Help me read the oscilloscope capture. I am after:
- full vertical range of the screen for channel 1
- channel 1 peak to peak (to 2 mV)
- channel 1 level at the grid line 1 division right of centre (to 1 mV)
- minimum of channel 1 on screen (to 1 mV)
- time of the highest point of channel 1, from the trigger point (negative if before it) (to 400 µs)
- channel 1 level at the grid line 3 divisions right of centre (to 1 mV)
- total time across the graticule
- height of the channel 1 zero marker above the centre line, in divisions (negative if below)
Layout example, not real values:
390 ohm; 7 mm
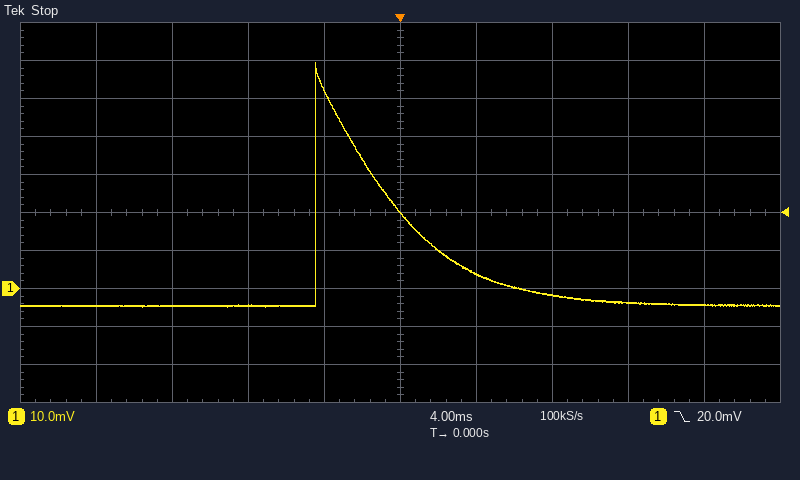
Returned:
100 mV; 64 mV; 4 mV; -5 mV; -4.4 ms; -4 mV; 40 ms; -2.0 div
